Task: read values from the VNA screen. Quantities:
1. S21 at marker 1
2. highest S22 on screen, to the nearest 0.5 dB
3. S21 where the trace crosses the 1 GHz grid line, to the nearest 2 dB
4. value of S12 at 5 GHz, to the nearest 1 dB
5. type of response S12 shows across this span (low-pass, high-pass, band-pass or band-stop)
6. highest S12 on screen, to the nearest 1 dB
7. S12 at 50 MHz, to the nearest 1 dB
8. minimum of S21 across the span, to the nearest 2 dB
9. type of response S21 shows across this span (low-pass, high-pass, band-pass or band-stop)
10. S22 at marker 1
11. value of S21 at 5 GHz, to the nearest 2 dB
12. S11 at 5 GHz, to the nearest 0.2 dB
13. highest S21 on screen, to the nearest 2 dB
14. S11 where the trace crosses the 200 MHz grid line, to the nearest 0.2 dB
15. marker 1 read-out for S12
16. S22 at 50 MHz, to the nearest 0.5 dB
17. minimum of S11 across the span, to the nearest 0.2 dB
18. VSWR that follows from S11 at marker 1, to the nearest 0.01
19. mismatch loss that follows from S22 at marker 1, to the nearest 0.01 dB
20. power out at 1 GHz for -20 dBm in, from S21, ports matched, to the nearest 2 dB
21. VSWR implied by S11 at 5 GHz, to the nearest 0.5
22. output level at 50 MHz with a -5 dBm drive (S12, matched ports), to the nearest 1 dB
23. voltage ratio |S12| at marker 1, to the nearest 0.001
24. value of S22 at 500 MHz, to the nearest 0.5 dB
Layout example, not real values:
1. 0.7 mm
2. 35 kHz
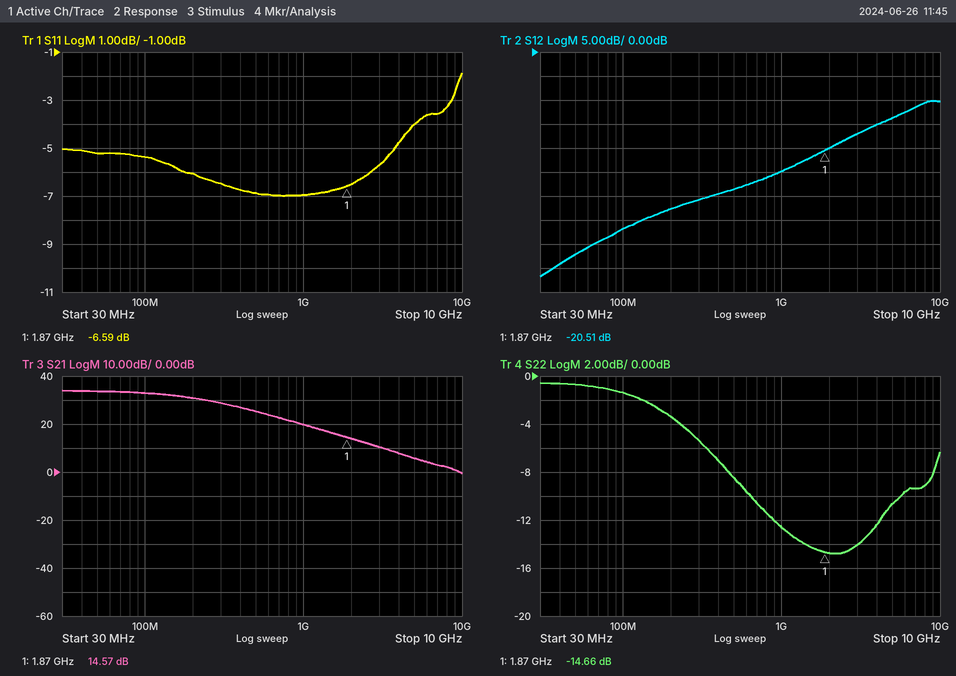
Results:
1. 14.57 dB
2. -0.5 dB
3. 20 dB
4. -14 dB
5. high-pass
6. -10 dB
7. -42 dB
8. 0 dB
9. low-pass
10. -14.66 dB
11. 6 dB
12. -4.0 dB
13. 34 dB
14. -6.0 dB
15. -20.51 dB
16. -0.5 dB
17. -7.0 dB
18. 2.76
19. 0.15 dB
20. 0 dBm
21. 4.5
22. -47 dBm
23. 0.094
24. -8.5 dB
